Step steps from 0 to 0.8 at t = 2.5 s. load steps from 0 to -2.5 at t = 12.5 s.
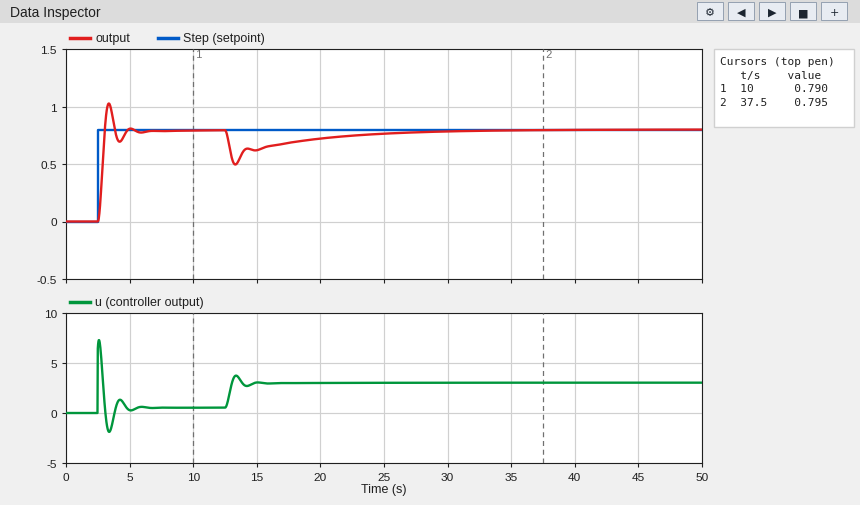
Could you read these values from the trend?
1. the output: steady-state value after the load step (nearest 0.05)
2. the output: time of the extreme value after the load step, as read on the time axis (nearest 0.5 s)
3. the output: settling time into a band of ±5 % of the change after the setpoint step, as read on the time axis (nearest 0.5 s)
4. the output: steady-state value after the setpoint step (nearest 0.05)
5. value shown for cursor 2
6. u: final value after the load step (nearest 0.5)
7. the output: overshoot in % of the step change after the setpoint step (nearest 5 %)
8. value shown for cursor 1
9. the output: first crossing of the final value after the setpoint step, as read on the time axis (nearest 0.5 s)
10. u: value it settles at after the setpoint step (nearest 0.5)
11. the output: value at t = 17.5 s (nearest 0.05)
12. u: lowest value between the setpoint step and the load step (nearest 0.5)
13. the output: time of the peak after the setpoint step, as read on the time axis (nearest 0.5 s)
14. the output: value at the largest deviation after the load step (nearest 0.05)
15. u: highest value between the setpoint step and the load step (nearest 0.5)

0.80
13.5 s
4.5 s
0.80
0.795
3.0
30 %
0.790
3.0 s
0.5
0.70
-2.0
3.5 s
0.50
7.5
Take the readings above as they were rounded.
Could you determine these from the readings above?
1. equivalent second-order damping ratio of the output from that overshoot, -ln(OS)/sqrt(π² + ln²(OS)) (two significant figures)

0.36
